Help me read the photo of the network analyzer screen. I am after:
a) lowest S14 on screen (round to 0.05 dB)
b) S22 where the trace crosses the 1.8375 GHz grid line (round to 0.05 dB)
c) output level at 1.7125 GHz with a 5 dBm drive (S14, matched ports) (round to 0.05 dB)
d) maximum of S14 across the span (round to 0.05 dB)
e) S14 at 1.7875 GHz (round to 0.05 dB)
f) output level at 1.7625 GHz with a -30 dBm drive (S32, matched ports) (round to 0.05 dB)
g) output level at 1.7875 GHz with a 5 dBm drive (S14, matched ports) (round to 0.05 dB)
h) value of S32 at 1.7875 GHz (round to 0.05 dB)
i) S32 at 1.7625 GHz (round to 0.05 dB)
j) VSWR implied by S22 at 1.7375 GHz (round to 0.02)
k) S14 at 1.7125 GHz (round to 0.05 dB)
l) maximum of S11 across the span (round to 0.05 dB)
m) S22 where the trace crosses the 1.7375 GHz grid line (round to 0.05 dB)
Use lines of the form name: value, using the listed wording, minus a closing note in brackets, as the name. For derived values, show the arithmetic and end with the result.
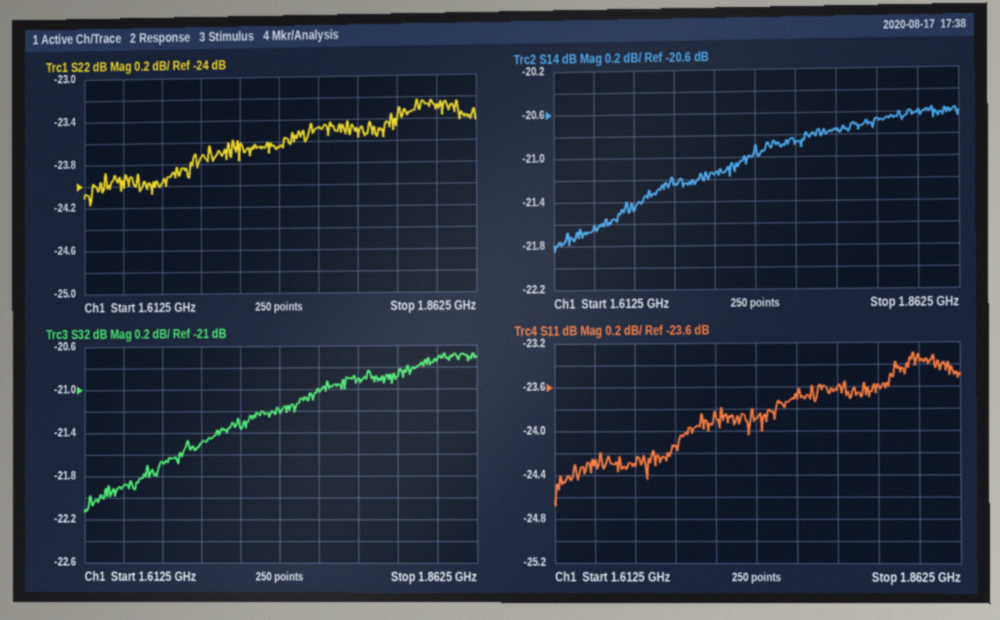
lowest S14 on screen: -21.85 dB
S22 where the trace crosses the 1.8375 GHz grid line: -23.30 dB
output level at 1.7125 GHz with a 5 dBm drive (S14, matched ports): 5 dBm + (-21.15 dB) = -16.15 dBm
maximum of S14 across the span: -20.55 dB
S14 at 1.7875 GHz: -20.75 dB
output level at 1.7625 GHz with a -30 dBm drive (S32, matched ports): -30 dBm + (-21.00 dB) = -51.00 dBm
output level at 1.7875 GHz with a 5 dBm drive (S14, matched ports): 5 dBm + (-20.75 dB) = -15.75 dBm
value of S32 at 1.7875 GHz: -20.90 dB
S32 at 1.7625 GHz: -21.00 dB
VSWR implied by S22 at 1.7375 GHz: |Γ| = 10^(-23.65/20) = 0.0657; VSWR = (1 + 0.0657)/(1 − 0.0657) ≈ 1.14
S14 at 1.7125 GHz: -21.15 dB
maximum of S11 across the span: -23.30 dB
S22 where the trace crosses the 1.7375 GHz grid line: -23.65 dB
